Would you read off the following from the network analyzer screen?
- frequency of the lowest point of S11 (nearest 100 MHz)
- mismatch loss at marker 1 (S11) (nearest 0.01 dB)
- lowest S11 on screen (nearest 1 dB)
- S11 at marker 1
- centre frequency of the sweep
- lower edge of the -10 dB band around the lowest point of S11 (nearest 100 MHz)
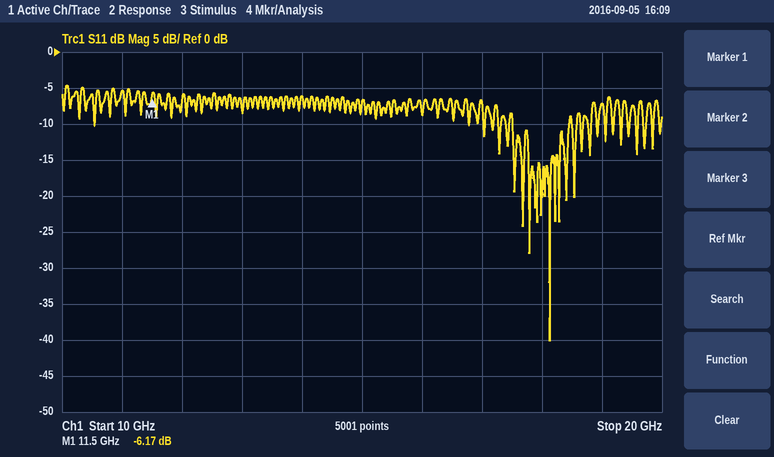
18.1 GHz
1.20 dB
-40 dB
-6.17 dB
15 GHz
17.5 GHz
